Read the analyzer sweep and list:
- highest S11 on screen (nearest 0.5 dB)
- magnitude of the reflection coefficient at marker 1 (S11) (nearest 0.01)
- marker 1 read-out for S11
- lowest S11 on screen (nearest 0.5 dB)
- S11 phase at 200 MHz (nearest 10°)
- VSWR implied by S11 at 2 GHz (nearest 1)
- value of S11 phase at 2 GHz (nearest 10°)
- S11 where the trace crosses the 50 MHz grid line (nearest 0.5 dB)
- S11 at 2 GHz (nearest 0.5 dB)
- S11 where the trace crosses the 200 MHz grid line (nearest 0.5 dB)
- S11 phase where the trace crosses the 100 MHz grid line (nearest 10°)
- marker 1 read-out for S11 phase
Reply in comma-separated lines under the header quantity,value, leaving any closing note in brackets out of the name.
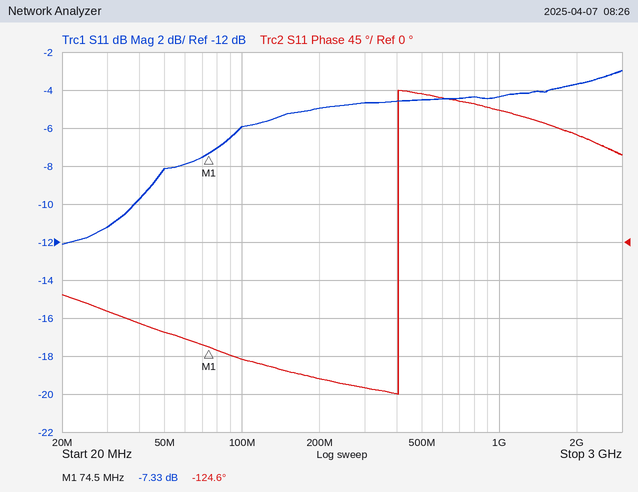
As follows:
quantity,value
highest S11 on screen,-3.0 dB
magnitude of the reflection coefficient at marker 1 (S11),0.43
marker 1 read-out for S11,-7.33 dB
lowest S11 on screen,-12.0 dB
S11 phase at 200 MHz,-160°
VSWR implied by S11 at 2 GHz,5
value of S11 phase at 2 GHz,130°
S11 where the trace crosses the 50 MHz grid line,-8.0 dB
S11 at 2 GHz,-3.5 dB
S11 where the trace crosses the 200 MHz grid line,-5.0 dB
S11 phase where the trace crosses the 100 MHz grid line,-140°
marker 1 read-out for S11 phase,-124.6°
